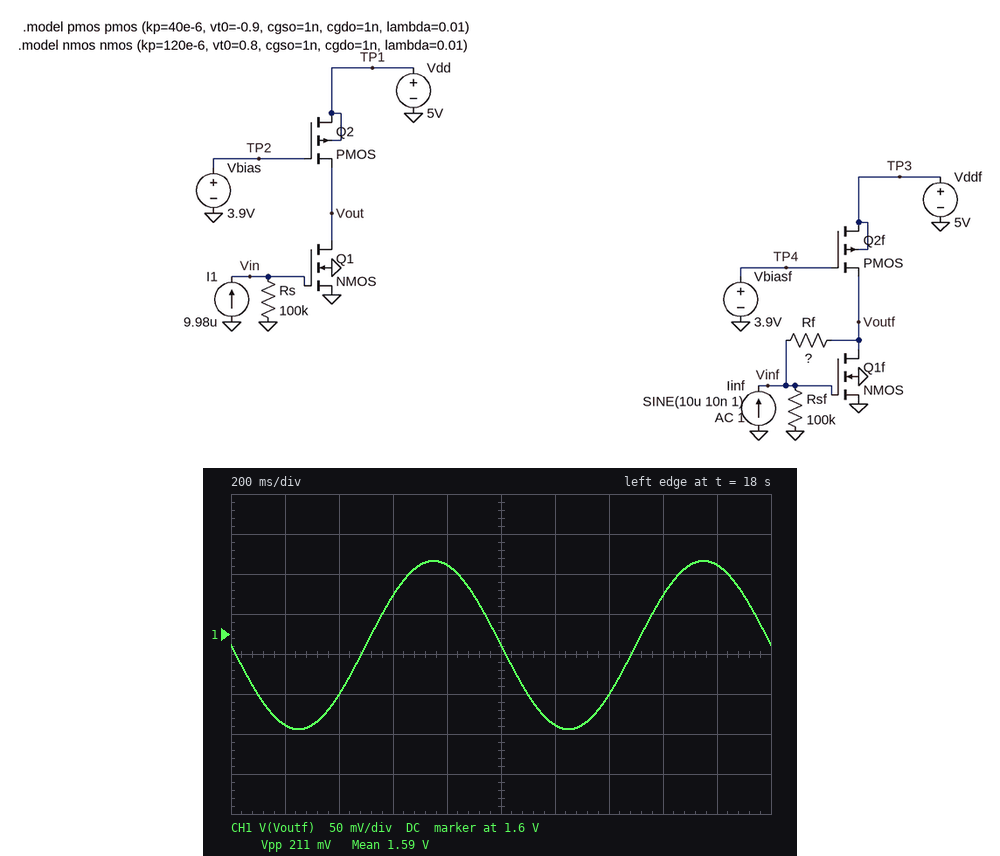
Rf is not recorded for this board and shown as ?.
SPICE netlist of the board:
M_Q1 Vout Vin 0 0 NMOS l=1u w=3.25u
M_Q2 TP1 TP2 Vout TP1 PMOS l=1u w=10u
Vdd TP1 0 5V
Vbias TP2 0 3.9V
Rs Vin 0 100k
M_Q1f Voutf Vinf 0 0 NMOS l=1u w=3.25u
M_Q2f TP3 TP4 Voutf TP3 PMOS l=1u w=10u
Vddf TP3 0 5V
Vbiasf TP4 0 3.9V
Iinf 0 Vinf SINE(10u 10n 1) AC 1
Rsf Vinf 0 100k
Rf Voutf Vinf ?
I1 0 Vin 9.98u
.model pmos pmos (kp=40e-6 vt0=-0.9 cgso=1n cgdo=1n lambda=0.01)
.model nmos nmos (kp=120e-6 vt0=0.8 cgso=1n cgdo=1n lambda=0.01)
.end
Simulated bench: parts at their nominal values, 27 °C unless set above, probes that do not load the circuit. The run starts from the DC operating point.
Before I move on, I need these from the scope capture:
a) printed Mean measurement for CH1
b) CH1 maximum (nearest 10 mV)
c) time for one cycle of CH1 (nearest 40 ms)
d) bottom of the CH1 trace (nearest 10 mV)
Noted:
1.59 V
1.69 V
1.00 s
1.48 V
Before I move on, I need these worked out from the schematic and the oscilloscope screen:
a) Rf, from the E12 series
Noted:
15 MΩ
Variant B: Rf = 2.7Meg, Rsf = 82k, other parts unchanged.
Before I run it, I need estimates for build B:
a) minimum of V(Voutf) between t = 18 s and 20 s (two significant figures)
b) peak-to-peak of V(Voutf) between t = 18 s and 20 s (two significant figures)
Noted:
4.9 V
1.9 mV
